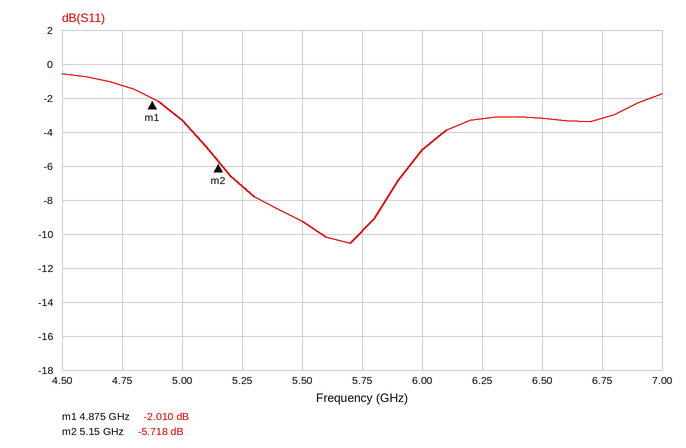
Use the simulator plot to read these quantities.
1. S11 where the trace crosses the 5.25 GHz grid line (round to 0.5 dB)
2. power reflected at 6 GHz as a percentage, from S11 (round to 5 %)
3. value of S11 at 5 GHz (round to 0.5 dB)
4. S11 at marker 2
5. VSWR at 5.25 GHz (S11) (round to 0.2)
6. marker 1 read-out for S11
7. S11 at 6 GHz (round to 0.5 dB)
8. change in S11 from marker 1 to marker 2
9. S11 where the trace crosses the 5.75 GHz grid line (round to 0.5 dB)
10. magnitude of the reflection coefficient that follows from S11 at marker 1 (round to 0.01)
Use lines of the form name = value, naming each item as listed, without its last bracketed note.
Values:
S11 where the trace crosses the 5.25 GHz grid line = -7.0 dB
power reflected at 6 GHz as a percentage, from S11 = 30 %
value of S11 at 5 GHz = -3.5 dB
S11 at marker 2 = -5.718 dB
VSWR at 5.25 GHz (S11) = 2.6
marker 1 read-out for S11 = -2.010 dB
S11 at 6 GHz = -5.0 dB
change in S11 from marker 1 to marker 2 = -3.708 dB
S11 where the trace crosses the 5.75 GHz grid line = -10.0 dB
magnitude of the reflection coefficient that follows from S11 at marker 1 = 0.79
